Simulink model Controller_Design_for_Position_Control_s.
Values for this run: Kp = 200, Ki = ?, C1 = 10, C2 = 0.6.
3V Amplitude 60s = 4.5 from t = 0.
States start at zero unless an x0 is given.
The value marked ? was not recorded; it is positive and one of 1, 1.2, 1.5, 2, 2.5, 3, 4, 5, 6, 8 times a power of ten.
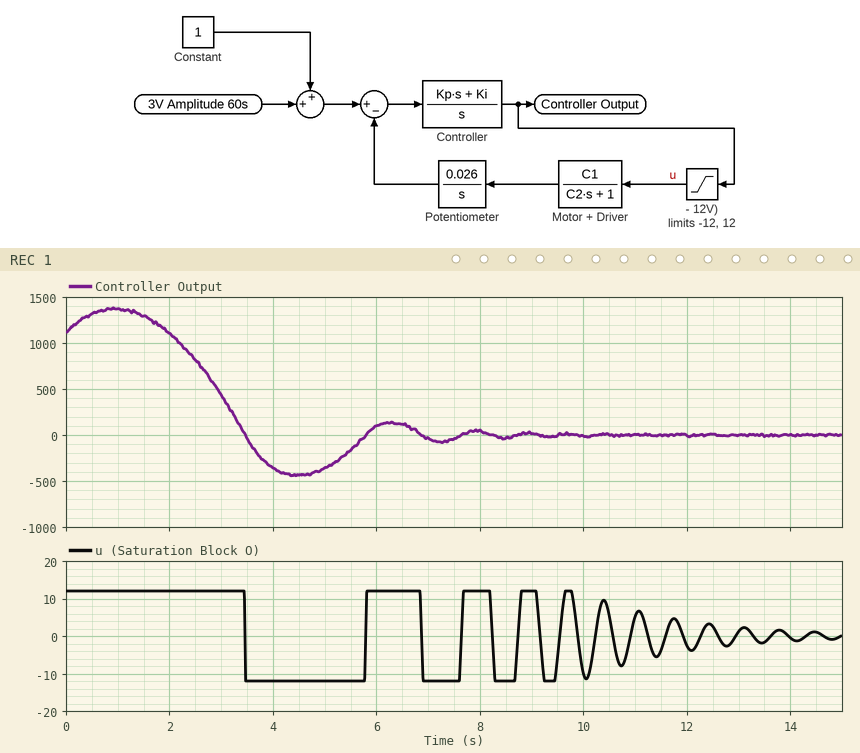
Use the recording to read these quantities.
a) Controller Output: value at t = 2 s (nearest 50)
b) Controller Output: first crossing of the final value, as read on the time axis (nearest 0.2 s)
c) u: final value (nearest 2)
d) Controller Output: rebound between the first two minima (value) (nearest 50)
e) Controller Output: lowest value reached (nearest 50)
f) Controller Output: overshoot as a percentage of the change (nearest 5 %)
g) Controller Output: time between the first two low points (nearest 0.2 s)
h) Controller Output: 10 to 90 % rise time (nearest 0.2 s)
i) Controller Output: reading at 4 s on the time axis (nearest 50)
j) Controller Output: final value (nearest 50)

1100
3.4 s
0
150
-450
40 %
2.8 s
1.2 s
-350
0
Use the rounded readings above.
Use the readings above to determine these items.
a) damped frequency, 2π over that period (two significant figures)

2.2 rad/s
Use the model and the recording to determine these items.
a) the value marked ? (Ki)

120
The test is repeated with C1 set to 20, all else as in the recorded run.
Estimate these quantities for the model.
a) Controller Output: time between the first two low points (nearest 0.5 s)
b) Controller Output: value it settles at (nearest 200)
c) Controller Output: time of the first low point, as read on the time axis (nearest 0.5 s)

2.0 s
0
2.5 s
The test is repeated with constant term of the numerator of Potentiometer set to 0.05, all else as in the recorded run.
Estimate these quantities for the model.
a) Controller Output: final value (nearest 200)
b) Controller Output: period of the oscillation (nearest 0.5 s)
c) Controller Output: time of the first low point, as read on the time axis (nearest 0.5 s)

0
2.0 s
2.5 s
